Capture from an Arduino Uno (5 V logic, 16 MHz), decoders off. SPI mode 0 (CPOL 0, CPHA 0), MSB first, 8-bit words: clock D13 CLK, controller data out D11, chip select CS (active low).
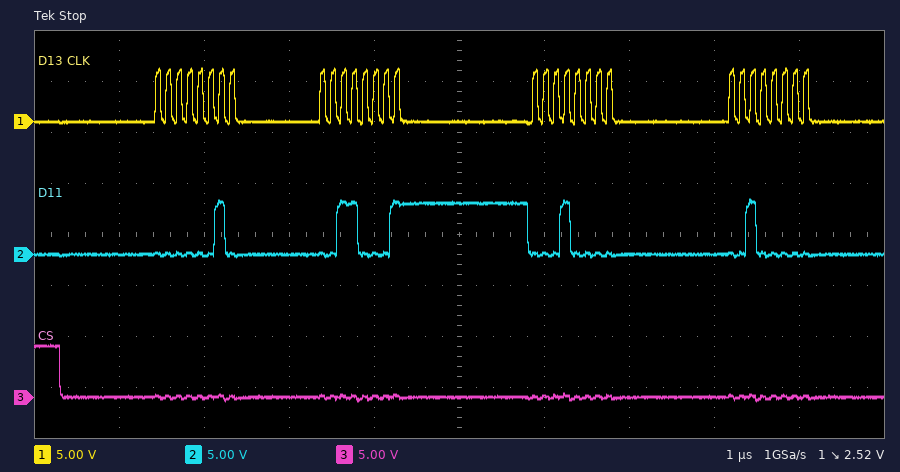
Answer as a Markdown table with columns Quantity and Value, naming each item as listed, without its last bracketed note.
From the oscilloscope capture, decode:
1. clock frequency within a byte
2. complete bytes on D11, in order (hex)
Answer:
| Quantity | Value |
|---|---|
| clock frequency within a byte | 8 MHz |
| complete bytes on D11, in order | 02 31 10 20 |
